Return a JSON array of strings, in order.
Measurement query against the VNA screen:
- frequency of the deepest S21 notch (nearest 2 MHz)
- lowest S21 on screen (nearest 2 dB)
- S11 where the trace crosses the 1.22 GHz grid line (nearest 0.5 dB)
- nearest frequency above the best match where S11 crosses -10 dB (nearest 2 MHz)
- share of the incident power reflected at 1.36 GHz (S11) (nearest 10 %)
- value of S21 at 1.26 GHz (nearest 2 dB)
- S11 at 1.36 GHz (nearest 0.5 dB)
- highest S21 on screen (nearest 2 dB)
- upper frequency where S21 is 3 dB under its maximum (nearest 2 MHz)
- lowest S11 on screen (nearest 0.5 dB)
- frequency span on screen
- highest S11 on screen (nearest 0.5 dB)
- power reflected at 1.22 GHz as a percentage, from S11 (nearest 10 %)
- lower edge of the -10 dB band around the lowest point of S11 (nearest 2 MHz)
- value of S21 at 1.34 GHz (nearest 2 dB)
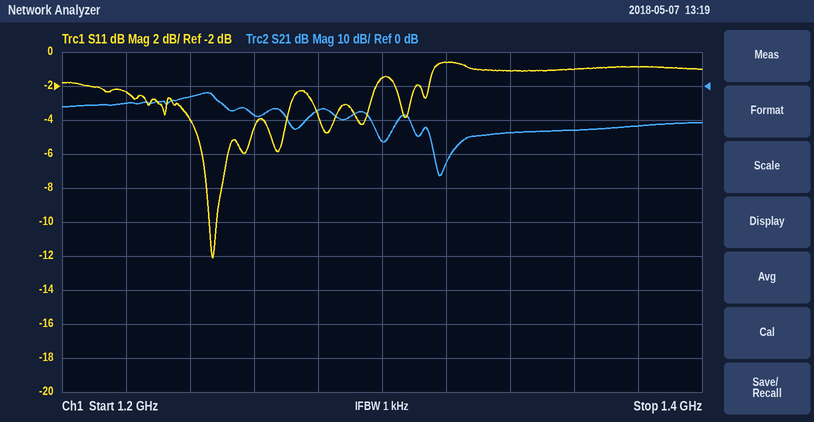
["1.318 GHz", "-26 dB", "-2.5 dB", "1.248 GHz", "80 %", "-8 dB", "-1.0 dB", "-2 dB", "1.250 GHz", "-12.0 dB", "200 MHz", "-0.5 dB", "60 %", "1.246 GHz", "-14 dB"]
